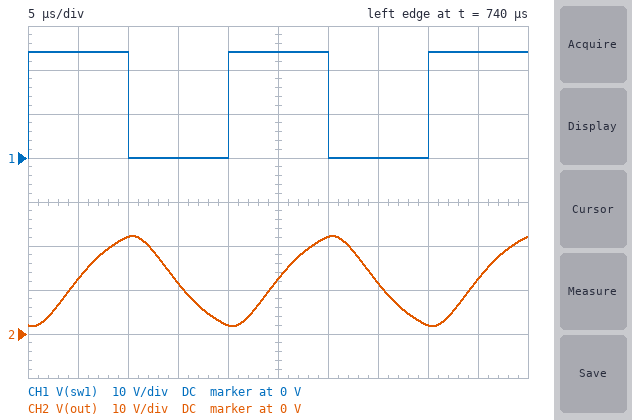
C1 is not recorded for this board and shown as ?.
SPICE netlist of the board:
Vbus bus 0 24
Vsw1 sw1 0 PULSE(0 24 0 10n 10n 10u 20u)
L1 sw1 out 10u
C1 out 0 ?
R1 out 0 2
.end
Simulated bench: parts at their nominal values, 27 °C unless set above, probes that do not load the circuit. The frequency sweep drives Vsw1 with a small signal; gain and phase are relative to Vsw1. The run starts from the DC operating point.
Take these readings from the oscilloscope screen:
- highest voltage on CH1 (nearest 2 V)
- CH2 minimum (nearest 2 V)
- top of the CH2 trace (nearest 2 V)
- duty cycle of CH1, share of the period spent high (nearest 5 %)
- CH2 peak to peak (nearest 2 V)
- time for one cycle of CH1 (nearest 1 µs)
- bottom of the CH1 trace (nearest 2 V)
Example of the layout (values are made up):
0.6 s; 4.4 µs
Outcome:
24 V; 2 V; 22 V; 50 %; 20 V; 20 µs; 0 V
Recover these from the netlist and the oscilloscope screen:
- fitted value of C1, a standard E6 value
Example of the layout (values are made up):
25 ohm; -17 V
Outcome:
1 µF
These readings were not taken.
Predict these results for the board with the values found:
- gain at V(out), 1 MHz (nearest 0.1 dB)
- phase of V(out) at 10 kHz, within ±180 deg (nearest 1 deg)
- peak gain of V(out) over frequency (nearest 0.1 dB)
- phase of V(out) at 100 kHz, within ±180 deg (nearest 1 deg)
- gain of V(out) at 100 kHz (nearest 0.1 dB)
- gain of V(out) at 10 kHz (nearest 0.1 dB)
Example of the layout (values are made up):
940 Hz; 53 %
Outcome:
-51.9 dB; -18 deg; 0 dB; -133 deg; -12.7 dB; -0.1 dB
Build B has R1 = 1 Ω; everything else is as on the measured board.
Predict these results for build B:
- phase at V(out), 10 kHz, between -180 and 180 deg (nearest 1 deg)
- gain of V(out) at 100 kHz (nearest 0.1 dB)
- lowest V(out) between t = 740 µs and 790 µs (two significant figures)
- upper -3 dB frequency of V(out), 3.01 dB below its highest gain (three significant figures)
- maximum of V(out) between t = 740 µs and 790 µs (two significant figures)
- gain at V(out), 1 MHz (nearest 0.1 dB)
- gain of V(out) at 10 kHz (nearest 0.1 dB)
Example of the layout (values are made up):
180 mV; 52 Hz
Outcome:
-33 deg; -16.8 dB; 6.6 V; 17.7 kHz; 17 V; -52.0 dB; -1.2 dB
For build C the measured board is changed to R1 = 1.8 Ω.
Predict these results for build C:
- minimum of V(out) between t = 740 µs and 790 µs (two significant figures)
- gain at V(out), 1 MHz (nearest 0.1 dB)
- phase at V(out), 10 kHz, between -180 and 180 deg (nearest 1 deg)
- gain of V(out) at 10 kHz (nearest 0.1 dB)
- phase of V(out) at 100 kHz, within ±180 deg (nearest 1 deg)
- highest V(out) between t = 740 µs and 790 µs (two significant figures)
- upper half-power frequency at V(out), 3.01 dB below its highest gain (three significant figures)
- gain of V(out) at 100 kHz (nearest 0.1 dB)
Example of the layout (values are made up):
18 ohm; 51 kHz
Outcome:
2.7 V; -51.9 dB; -20 deg; -0.2 dB; -130 deg; 21 V; 38.8 kHz; -13.2 dB
